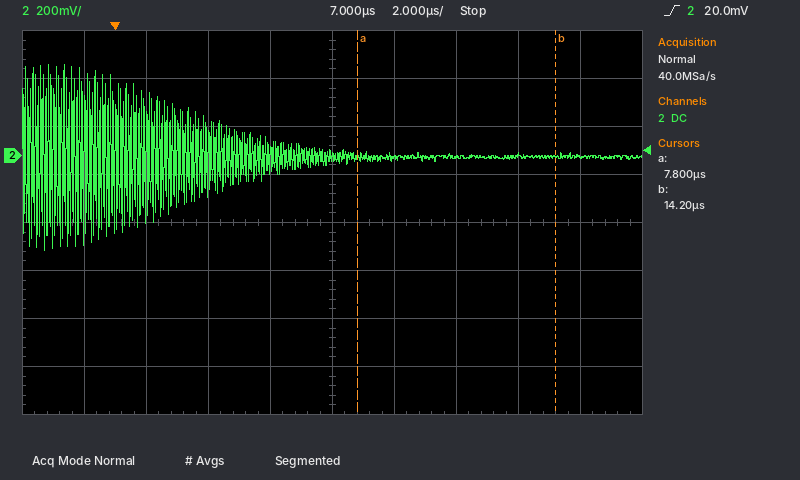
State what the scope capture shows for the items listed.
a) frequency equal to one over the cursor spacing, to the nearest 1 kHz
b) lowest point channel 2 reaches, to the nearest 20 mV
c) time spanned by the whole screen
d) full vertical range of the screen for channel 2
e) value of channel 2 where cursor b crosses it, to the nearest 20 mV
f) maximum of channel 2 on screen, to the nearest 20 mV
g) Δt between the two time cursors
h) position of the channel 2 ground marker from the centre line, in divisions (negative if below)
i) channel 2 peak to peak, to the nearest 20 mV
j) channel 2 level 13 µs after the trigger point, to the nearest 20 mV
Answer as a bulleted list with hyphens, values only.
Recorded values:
- 156 kHz
- -400 mV
- 20 µs
- 1.6 V
- 0 mV
- 380 mV
- 6.4 µs
- +1.4 div
- 780 mV
- 0 mV
